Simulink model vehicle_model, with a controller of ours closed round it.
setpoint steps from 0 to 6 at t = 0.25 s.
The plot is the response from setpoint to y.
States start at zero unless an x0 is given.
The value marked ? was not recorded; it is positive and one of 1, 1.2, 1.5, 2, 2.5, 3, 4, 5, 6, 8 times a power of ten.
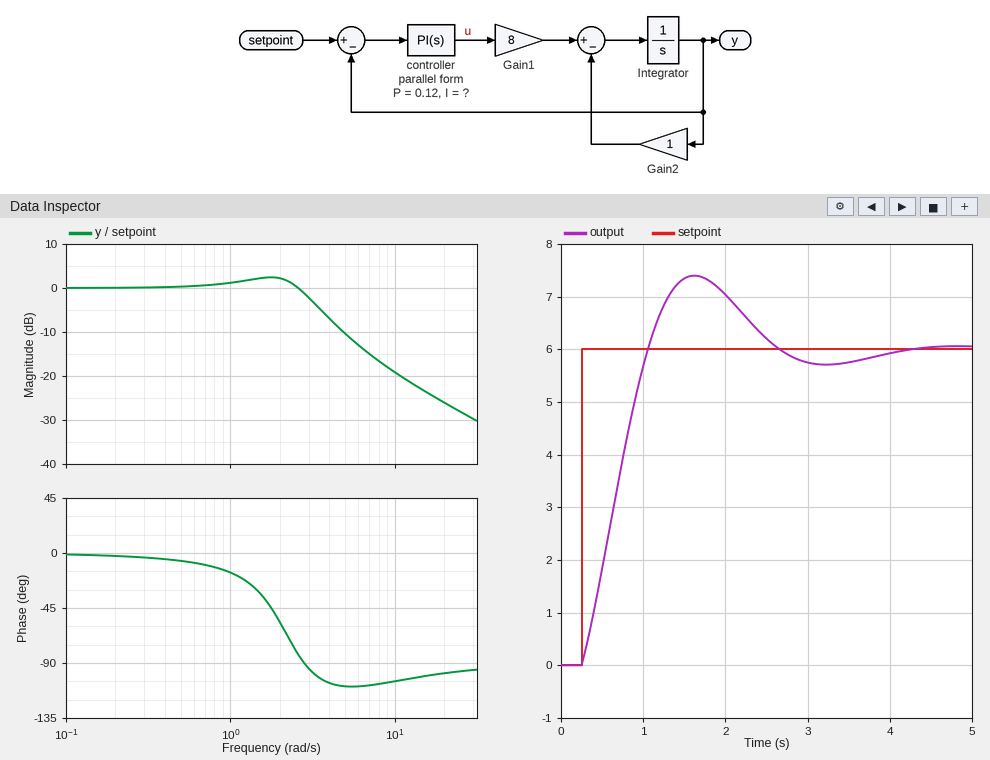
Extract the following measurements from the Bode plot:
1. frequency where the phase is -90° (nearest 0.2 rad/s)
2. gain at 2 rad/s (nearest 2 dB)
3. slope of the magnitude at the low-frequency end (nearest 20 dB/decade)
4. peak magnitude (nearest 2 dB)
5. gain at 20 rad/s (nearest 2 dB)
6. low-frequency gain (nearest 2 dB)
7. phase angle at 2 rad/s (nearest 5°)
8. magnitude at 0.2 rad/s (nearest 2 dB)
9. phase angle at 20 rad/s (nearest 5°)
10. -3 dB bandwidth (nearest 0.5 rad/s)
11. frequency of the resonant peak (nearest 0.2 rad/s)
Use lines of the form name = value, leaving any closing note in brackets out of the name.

frequency where the phase is -90° = 2.8 rad/s
gain at 2 rad/s = 2 dB
slope of the magnitude at the low-frequency end = 0 dB/decade
peak magnitude = 2 dB
gain at 20 rad/s = -26 dB
low-frequency gain = 0 dB
phase angle at 2 rad/s = -55°
magnitude at 0.2 rad/s = 0 dB
phase angle at 20 rad/s = -100°
-3 dB bandwidth = 3.0 rad/s
frequency of the resonant peak = 1.8 rad/s
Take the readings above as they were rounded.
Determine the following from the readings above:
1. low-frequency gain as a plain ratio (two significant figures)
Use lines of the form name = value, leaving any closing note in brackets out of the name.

low-frequency gain as a plain ratio = 1.0
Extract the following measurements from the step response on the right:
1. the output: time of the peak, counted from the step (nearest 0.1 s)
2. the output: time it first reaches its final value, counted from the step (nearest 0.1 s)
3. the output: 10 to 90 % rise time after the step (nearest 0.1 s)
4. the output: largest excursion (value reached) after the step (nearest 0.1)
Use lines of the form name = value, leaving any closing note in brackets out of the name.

the output: time of the peak, counted from the step = 1.4 s
the output: time it first reaches its final value, counted from the step = 0.8 s
the output: 10 to 90 % rise time after the step = 0.6 s
the output: largest excursion (value reached) after the step = 7.4
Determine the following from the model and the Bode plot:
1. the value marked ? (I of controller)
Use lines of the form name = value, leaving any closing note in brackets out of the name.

the value marked ? = 0.6
